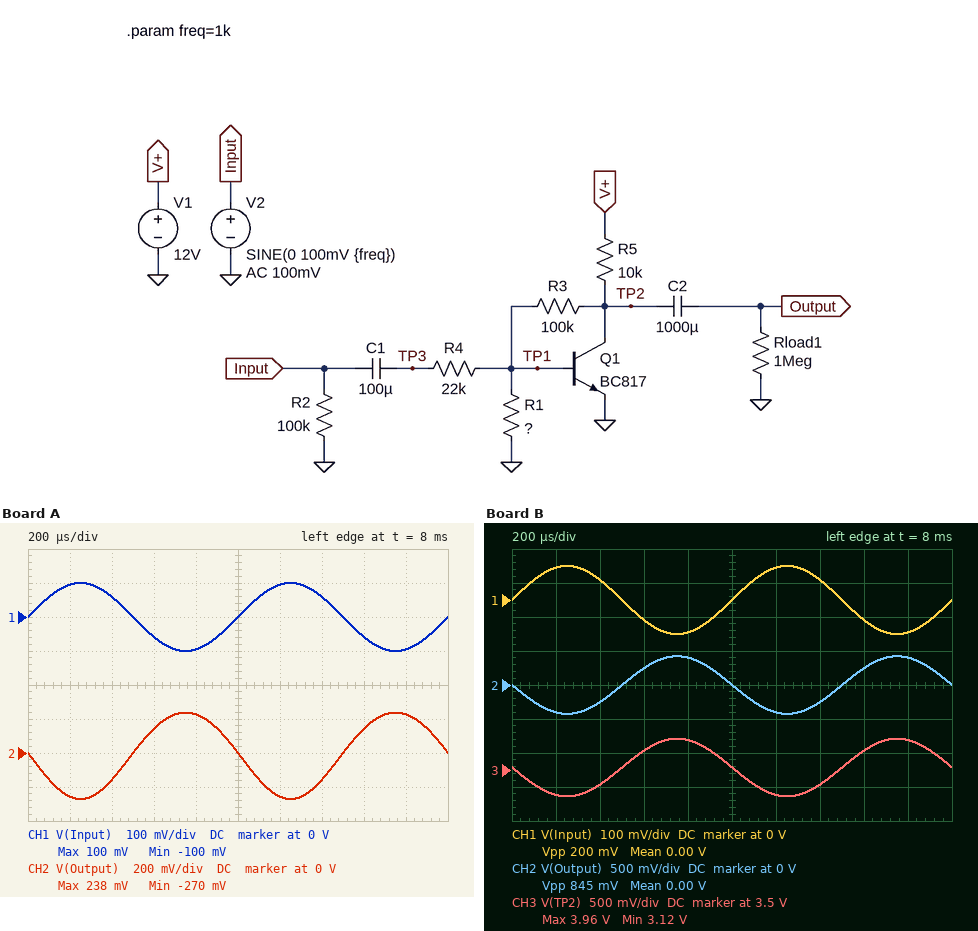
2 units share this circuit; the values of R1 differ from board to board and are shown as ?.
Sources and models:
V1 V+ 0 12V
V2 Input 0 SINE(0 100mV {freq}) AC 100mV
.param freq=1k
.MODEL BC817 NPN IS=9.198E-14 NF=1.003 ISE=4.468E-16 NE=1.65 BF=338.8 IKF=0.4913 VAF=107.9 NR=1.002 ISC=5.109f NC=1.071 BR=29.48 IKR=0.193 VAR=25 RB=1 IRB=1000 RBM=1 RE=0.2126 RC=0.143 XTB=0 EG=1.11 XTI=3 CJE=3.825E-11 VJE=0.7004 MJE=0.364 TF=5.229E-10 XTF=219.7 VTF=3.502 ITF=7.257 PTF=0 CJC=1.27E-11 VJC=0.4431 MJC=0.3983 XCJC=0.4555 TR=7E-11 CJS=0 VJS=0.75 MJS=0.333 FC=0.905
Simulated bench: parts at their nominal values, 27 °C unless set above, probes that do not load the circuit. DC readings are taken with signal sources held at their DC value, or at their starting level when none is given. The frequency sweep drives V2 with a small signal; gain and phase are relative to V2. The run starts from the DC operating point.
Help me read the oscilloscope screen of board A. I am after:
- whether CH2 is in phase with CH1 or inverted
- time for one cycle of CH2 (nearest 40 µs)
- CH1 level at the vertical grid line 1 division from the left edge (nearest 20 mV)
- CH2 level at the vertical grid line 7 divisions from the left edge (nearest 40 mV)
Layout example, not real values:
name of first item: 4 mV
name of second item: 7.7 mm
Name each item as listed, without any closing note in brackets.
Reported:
whether CH2 is in phase with CH1 or inverted: inverted
time for one cycle of CH2: 1.00 ms
CH1 level at the vertical grid line 1 division from the left edge: 100 mV
CH2 level at the vertical grid line 7 divisions from the left edge: -160 mV
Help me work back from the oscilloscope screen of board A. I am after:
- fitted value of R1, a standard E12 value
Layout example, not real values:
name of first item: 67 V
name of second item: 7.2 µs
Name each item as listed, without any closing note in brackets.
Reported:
fitted value of R1, a standard E12 value: 5.6 kΩ
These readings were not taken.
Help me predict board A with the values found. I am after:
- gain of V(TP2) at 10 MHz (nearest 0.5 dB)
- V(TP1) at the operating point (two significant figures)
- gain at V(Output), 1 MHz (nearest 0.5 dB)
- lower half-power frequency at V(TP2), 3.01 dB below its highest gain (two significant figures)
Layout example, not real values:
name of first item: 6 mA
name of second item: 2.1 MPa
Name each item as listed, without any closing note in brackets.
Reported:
gain of V(TP2) at 10 MHz: -20.0 dB
V(TP1) at the operating point: 540 mV
gain at V(Output), 1 MHz: 1.0 dB
lower half-power frequency at V(TP2), 3.01 dB below its highest gain: 66 mHz
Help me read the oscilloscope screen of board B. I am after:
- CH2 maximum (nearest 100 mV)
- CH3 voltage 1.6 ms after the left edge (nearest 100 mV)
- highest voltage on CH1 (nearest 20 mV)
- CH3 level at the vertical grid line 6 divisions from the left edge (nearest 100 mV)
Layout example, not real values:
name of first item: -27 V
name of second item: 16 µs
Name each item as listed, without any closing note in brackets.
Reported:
CH2 maximum: 400 mV
CH3 voltage 1.6 ms after the left edge: 3.8 V
highest voltage on CH1: 100 mV
CH3 level at the vertical grid line 6 divisions from the left edge: 3.1 V
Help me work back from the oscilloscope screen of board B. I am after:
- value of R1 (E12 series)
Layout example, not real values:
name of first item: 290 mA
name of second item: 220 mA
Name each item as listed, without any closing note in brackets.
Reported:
value of R1: 22 kΩ
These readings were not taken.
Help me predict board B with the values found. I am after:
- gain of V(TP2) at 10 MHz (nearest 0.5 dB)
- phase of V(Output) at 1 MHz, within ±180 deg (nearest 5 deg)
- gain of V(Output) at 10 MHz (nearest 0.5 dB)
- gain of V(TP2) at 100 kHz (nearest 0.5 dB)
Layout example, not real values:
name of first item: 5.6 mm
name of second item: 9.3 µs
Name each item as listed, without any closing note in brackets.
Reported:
gain of V(TP2) at 10 MHz: -18.5 dB
phase of V(Output) at 1 MHz, within ±180 deg: 105 deg
gain of V(Output) at 10 MHz: -18.5 dB
gain of V(TP2) at 100 kHz: 12.0 dB
